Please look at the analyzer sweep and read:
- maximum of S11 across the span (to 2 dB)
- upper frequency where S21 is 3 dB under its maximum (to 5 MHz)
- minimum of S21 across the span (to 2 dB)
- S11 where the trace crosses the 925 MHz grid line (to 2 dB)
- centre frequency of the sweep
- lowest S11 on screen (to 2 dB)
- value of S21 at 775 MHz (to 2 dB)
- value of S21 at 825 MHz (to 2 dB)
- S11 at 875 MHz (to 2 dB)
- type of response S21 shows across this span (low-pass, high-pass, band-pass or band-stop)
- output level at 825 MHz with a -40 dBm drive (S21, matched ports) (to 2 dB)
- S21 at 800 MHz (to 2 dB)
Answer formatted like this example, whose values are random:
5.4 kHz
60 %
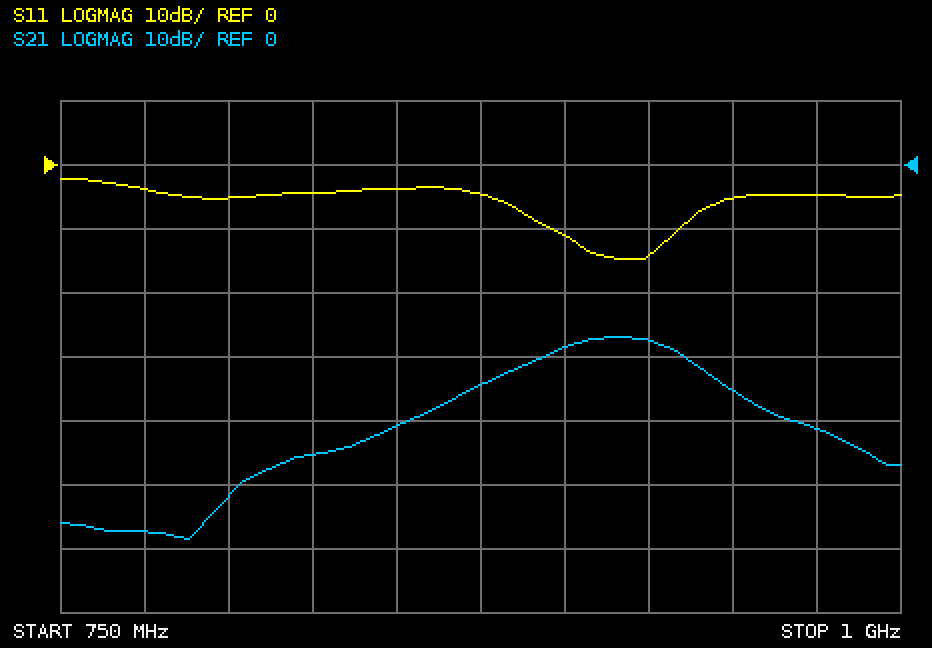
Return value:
-2 dB
935 MHz
-58 dB
-14 dB
875 MHz
-14 dB
-58 dB
-46 dB
-4 dB
band-pass
-86 dBm
-52 dB
